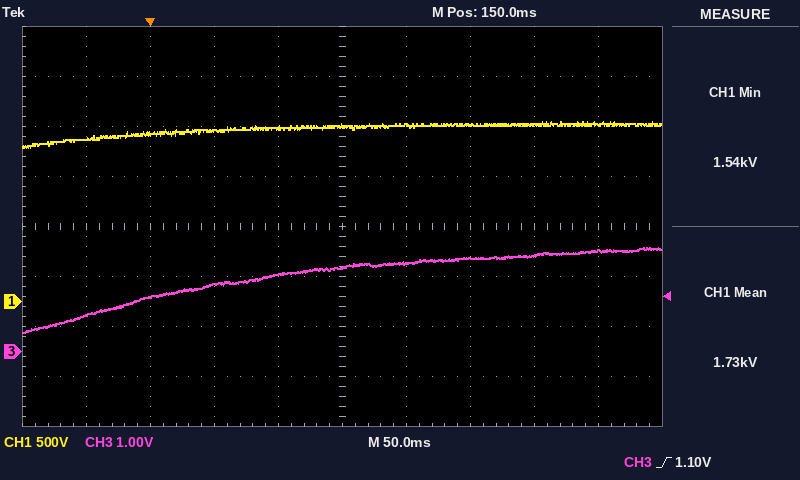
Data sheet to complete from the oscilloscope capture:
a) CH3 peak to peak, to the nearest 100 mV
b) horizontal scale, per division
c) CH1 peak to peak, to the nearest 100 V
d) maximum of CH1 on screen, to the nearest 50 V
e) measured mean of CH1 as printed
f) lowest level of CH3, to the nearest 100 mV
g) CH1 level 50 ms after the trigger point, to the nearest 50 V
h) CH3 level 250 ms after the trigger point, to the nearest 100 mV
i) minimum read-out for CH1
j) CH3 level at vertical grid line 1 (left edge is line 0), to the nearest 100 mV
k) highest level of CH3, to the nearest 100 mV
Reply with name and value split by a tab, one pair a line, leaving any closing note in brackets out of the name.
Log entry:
CH3 peak to peak, to the nearest 100 mV	1.7 V
horizontal scale, per division	50 ms
CH1 peak to peak, to the nearest 100 V	300 V
maximum of CH1 on screen, to the nearest 50 V	1.80 kV
measured mean of CH1 as printed	1.73 kV
lowest level of CH3, to the nearest 100 mV	400 mV
CH1 level 50 ms after the trigger point, to the nearest 50 V	1.70 kV
CH3 level 250 ms after the trigger point, to the nearest 100 mV	1.9 V
minimum read-out for CH1	1.54 kV
CH3 level at vertical grid line 1 (left edge is line 0), to the nearest 100 mV	700 mV
highest level of CH3, to the nearest 100 mV	2.1 V
